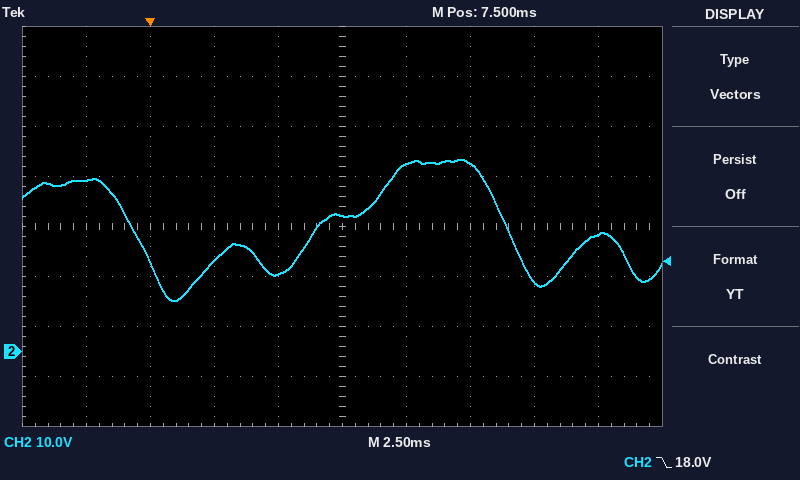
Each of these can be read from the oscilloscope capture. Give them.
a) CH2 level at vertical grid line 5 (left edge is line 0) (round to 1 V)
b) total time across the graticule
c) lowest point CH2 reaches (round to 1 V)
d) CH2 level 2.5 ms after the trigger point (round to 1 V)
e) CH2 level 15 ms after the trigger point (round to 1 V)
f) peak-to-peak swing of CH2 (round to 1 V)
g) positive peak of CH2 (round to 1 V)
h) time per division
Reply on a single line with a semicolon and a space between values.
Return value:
27 V; 25 ms; 10 V; 18 V; 14 V; 28 V; 38 V; 2.5 ms
